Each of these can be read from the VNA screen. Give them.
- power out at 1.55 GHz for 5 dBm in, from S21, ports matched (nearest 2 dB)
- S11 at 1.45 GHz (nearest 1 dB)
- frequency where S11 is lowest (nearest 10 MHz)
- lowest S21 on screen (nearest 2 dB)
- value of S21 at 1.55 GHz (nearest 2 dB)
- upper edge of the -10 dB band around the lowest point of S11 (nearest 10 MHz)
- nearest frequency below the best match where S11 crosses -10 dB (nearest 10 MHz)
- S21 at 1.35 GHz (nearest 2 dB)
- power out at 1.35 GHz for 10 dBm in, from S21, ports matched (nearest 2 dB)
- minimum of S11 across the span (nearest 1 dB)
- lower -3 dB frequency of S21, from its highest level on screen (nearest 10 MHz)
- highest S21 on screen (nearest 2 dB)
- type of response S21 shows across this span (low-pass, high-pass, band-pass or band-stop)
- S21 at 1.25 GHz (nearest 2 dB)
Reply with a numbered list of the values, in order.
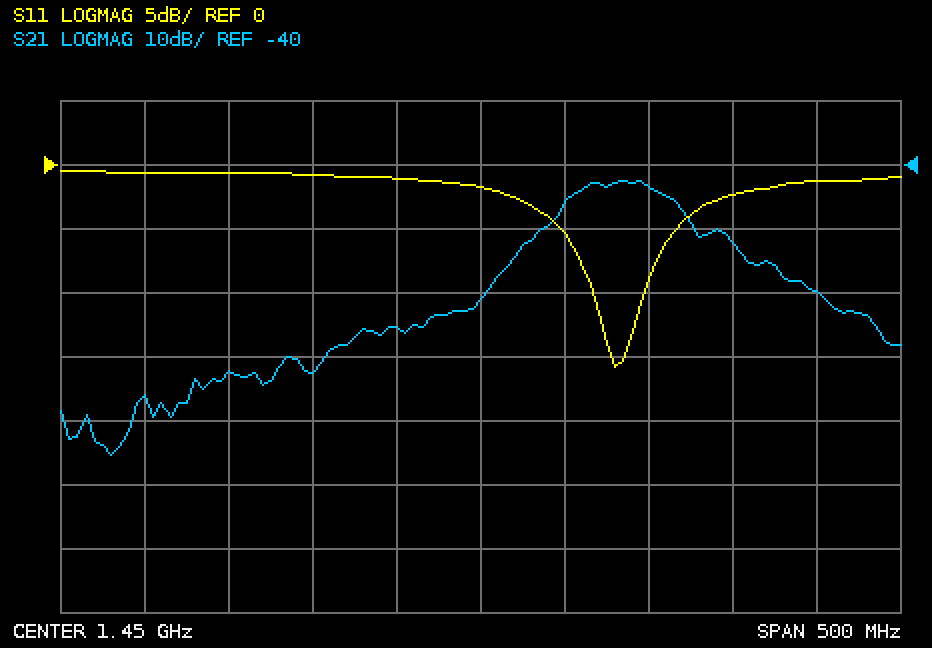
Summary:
1. -38 dBm
2. -2 dB
3. 1.53 GHz
4. -86 dB
5. -44 dB
6. 1.55 GHz
7. 1.52 GHz
8. -72 dB
9. -62 dBm
10. -16 dB
11. 1.50 GHz
12. -42 dB
13. band-pass
14. -76 dB
